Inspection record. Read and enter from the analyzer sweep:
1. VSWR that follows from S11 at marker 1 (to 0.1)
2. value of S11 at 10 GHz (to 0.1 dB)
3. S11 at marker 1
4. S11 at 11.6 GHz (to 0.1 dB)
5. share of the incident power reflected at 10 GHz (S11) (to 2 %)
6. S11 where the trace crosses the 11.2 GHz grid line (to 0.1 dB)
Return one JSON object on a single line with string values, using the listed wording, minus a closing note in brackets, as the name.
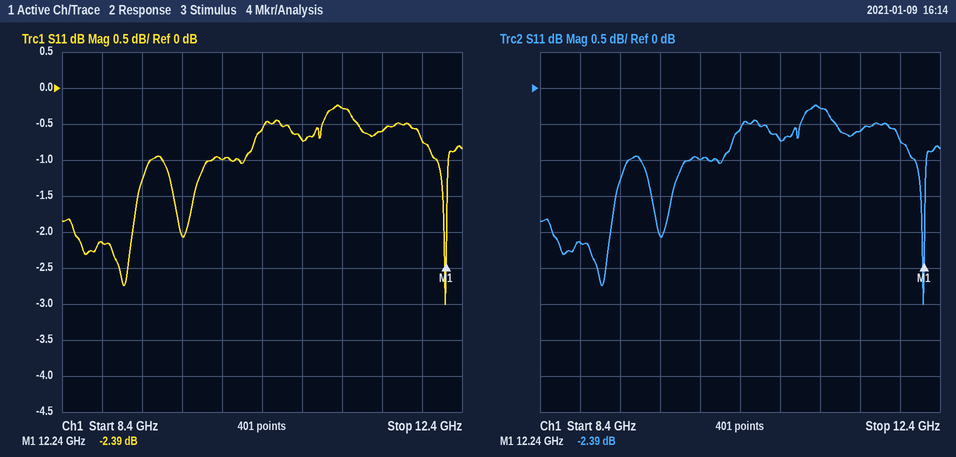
{"VSWR that follows from S11 at marker 1": "7.3", "value of S11 at 10 GHz": "-1.0 dB", "S11 at marker 1": "-2.39 dB", "S11 at 11.6 GHz": "-0.6 dB", "share of the incident power reflected at 10 GHz (S11)": "80 %", "S11 where the trace crosses the 11.2 GHz grid line": "-0.3 dB"}
